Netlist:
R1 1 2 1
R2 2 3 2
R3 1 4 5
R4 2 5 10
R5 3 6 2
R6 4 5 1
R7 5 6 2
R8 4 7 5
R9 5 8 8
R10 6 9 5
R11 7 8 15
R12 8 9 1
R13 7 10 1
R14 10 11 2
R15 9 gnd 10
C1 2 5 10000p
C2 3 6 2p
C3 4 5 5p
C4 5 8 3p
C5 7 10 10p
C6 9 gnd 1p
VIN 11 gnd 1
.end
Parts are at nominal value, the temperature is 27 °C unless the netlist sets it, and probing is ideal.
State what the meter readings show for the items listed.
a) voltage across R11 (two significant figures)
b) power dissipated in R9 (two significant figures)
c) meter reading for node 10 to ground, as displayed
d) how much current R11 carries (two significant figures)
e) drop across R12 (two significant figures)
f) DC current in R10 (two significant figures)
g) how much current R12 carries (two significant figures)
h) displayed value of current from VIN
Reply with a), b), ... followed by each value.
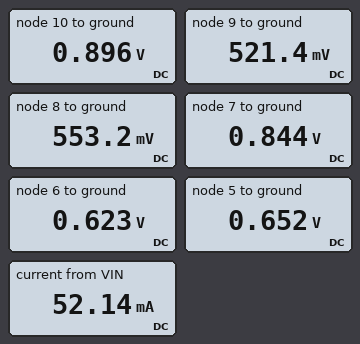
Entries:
a) 290 mV
b) 1.2 mW
c) 0.896 V
d) 19 mA
e) 32 mV
f) 20 mA
g) 32 mA
h) 52.14 mA
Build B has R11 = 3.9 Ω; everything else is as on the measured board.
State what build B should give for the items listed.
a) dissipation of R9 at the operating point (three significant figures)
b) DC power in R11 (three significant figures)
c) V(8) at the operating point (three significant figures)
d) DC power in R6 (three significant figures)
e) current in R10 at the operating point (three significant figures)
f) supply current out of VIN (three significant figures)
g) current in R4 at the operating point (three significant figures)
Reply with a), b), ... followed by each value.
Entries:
a) 252 µW
b) 6.60 mW
c) 657 mV
d) 267 µW
e) 14.2 mA
f) 61.0 mA
g) 466 µA
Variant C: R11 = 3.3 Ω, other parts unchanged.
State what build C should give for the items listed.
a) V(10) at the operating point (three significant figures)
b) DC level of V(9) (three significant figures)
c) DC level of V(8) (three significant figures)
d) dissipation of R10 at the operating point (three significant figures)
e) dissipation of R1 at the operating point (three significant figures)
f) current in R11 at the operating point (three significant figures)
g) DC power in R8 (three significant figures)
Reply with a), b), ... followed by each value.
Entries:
a) 876 mV
b) 621 mV
c) 669 mV
d) 908 µW
e) 10.7 µW
f) 43.8 mA
g) 1.67 mW
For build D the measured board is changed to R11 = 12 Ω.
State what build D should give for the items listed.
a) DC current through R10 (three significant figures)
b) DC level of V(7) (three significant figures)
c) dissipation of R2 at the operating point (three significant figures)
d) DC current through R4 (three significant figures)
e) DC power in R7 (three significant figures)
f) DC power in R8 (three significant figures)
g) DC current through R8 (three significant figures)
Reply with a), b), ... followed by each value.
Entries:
a) 19.5 mA
b) 840 mV
c) 63.7 µW
d) 509 µA
e) 383 µW
f) 4.76 mW
g) 30.9 mA
